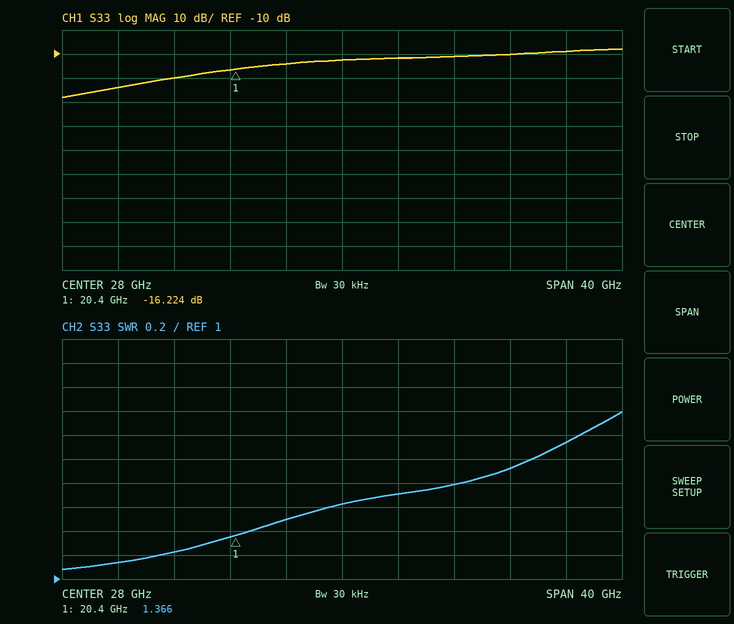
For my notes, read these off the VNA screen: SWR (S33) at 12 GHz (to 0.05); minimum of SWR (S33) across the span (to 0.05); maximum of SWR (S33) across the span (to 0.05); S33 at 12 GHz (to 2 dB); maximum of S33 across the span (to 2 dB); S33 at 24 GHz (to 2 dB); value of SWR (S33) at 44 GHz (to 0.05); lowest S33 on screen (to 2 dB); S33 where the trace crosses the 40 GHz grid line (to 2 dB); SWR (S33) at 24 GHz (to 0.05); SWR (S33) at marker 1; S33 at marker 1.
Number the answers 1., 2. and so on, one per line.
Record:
1. 1.15
2. 1.10
3. 2.40
4. -24 dB
5. -8 dB
6. -14 dB
7. 2.15
8. -28 dB
9. -10 dB
10. 1.50
11. 1.366
12. -16.224 dB
